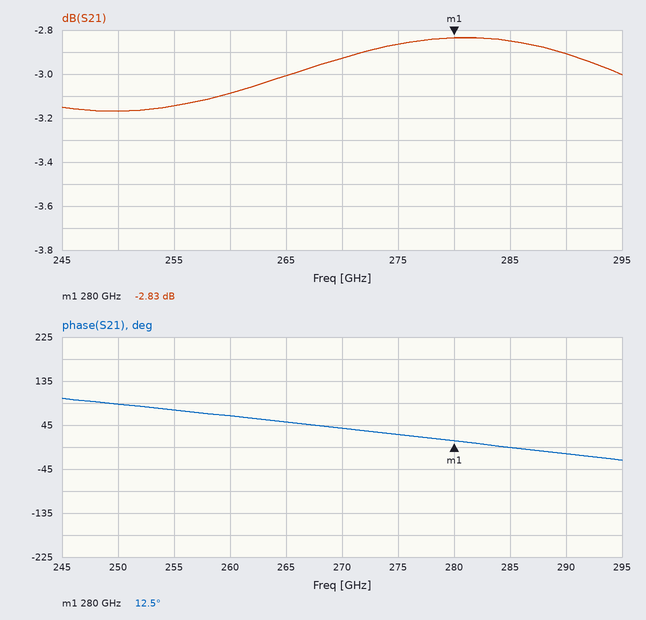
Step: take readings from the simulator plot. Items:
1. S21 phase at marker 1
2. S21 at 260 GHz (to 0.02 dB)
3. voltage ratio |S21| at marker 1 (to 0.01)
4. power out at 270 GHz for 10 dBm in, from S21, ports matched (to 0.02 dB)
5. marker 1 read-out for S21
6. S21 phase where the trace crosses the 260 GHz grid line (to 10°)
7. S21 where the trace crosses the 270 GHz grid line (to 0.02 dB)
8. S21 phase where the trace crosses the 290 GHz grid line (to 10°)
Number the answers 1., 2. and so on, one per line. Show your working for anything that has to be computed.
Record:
1. 12.5°
2. -3.08 dB
3. 10^(-2.83/20) ≈ 0.72
4. 10 dBm + (-2.92 dB) = 7.08 dBm
5. -2.83 dB
6. 60°
7. -2.92 dB
8. -10°
